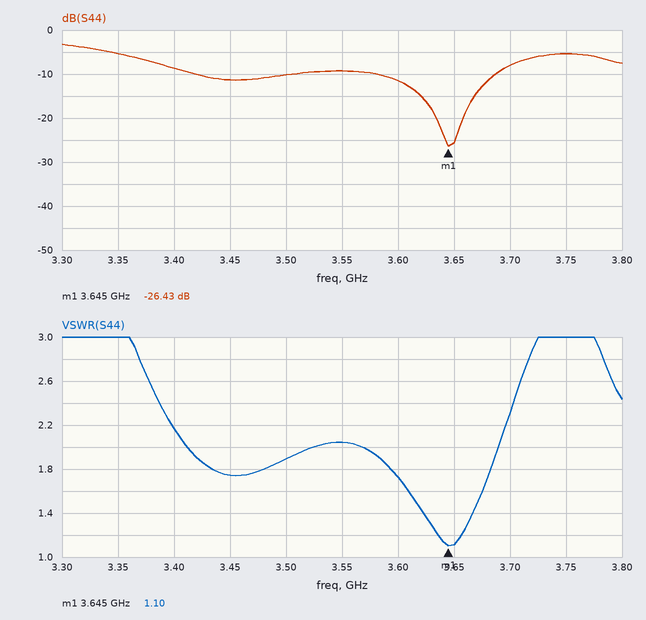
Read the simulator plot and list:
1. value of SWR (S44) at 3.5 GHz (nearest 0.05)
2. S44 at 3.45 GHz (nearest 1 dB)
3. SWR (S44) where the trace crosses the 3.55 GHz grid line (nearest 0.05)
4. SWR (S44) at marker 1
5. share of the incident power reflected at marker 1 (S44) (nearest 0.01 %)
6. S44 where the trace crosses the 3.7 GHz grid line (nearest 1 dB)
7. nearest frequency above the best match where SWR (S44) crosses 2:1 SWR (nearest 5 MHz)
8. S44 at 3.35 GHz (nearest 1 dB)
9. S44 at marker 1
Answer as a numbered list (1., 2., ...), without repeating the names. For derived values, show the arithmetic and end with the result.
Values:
1. 1.90
2. -11 dB
3. 2.05
4. 1.10
5. 10^(-26.43/10) ≈ 0.23 %
6. -8 dB
7. 3.690 GHz
8. -5 dB
9. -26.43 dB
